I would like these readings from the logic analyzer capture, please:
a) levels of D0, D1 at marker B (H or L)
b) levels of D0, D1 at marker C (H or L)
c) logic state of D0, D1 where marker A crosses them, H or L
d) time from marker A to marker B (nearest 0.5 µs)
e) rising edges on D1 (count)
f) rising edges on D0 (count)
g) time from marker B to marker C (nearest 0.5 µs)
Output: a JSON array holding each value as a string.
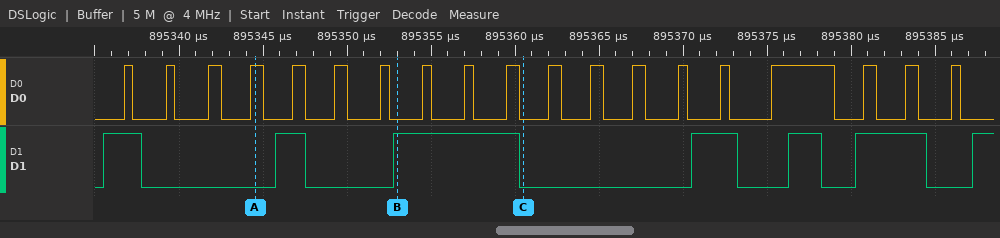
["D0=L, D1=H", "D0=L, D1=L", "D0=H, D1=L", "8.5 µs", "7", "19", "7.5 µs"]
